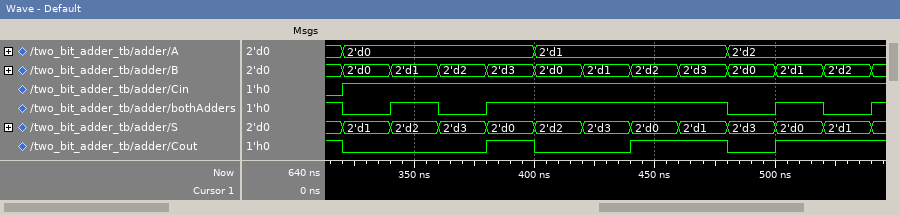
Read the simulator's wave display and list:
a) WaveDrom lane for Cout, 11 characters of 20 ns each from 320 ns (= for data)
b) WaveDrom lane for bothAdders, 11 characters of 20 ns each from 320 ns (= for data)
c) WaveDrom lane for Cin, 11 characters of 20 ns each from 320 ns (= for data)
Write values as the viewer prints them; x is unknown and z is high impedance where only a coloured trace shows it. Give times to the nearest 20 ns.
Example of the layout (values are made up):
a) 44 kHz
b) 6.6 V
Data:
a) {name: 'Cout', wave: '0..10.1.01.'}
b) {name: 'bothAdders', wave: '0101....010'}
c) {name: 'Cin', wave: '1..........'}
